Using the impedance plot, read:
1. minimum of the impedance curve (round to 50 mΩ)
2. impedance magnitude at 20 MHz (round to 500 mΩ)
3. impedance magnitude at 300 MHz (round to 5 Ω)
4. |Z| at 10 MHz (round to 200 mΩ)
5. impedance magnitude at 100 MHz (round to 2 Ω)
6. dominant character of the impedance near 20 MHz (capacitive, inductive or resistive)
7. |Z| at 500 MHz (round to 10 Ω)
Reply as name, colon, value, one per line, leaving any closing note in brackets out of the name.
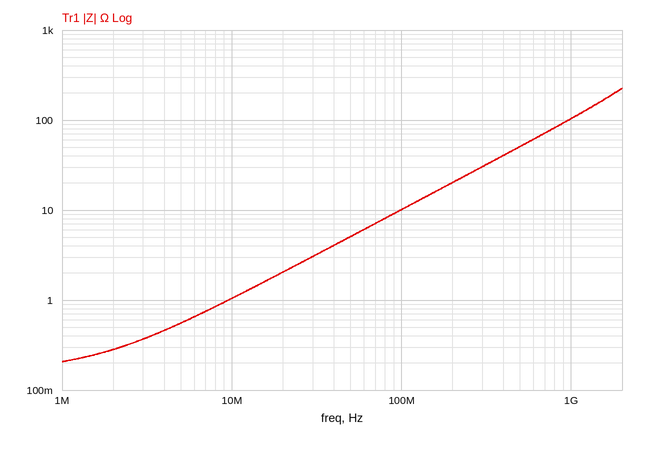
minimum of the impedance curve: 200 mΩ
impedance magnitude at 20 MHz: 2.0 Ω
impedance magnitude at 300 MHz: 30 Ω
|Z| at 10 MHz: 1.0 Ω
impedance magnitude at 100 MHz: 10 Ω
dominant character of the impedance near 20 MHz: inductive
|Z| at 500 MHz: 50 Ω
